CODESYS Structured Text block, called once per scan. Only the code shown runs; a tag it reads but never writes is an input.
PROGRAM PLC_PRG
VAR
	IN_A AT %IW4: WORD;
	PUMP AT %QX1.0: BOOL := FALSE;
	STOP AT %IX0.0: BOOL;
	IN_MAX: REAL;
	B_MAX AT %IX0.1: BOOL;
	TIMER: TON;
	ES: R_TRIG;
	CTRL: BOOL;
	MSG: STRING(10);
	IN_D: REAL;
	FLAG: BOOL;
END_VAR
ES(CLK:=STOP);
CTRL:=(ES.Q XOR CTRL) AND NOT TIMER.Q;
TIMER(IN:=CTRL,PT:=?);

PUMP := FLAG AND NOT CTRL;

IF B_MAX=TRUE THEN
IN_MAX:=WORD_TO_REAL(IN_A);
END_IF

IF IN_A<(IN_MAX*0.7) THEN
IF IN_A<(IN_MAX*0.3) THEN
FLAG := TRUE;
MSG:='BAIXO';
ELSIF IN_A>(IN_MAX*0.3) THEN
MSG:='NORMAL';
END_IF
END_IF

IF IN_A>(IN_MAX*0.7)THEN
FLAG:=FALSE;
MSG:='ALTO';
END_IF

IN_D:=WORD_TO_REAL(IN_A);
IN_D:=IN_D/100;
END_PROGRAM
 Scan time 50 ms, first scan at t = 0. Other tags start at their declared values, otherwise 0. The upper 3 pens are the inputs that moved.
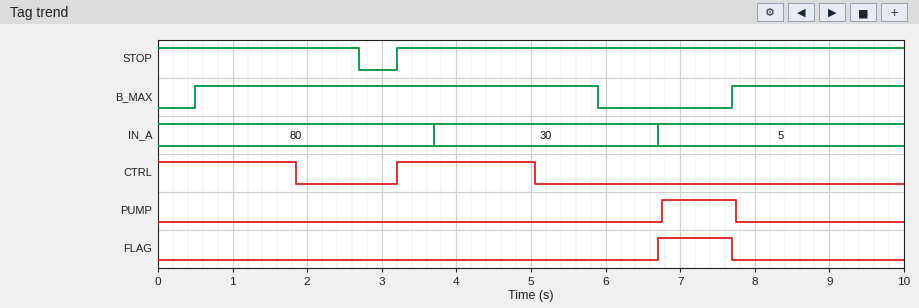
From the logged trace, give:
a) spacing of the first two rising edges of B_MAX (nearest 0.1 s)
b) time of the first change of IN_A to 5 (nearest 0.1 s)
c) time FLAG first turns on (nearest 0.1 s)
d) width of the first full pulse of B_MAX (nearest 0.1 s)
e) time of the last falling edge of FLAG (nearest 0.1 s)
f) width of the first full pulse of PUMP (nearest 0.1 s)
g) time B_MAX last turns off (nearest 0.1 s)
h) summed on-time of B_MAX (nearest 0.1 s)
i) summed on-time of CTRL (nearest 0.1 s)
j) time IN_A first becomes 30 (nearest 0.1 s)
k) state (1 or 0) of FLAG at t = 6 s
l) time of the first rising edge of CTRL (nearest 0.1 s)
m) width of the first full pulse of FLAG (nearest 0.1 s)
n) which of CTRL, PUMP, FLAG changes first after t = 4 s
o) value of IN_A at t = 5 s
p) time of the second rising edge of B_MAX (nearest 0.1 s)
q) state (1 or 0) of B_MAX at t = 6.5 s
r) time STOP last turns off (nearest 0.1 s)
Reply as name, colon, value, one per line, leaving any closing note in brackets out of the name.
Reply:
spacing of the first two rising edges of B_MAX: 7.2 s
time of the first change of IN_A to 5: 6.7 s
time FLAG first turns on: 6.7 s
width of the first full pulse of B_MAX: 5.4 s
time of the last falling edge of FLAG: 7.7 s
width of the first full pulse of PUMP: 1.0 s
time B_MAX last turns off: 5.9 s
summed on-time of B_MAX: 7.7 s
summed on-time of CTRL: 3.7 s
time IN_A first becomes 30: 3.7 s
state (1 or 0) of FLAG at t = 6 s: 0
time of the first rising edge of CTRL: 3.2 s
width of the first full pulse of FLAG: 1.0 s
which of CTRL, PUMP, FLAG changes first after t = 4 s: CTRL
value of IN_A at t = 5 s: 30
time of the second rising edge of B_MAX: 7.7 s
state (1 or 0) of B_MAX at t = 6.5 s: 0
time STOP last turns off: 2.7 s
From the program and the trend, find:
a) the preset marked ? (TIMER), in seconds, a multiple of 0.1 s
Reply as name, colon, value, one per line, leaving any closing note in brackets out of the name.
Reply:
the preset marked ? (TIMER), in seconds, a multiple of 0.1 s: 1.8 s
